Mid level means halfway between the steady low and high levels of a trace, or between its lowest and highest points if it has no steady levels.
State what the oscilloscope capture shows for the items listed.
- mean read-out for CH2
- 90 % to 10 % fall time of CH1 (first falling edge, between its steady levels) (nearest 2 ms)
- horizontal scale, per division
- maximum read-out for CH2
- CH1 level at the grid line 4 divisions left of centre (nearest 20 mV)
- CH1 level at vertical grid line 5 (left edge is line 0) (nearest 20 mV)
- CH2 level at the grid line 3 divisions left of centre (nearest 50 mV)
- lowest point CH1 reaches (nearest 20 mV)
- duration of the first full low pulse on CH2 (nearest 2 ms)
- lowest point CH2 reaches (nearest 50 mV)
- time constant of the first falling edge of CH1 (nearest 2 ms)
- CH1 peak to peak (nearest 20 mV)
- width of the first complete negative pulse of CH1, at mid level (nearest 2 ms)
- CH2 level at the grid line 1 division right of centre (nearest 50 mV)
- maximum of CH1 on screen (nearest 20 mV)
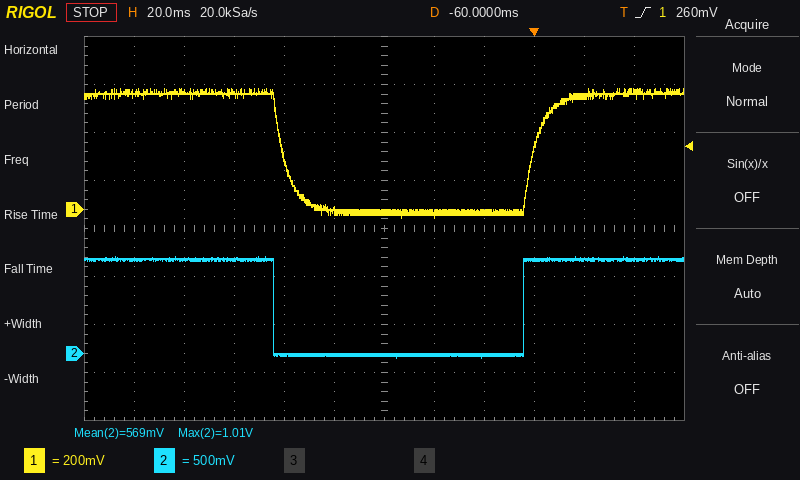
569 mV
12 ms
20 ms
1.01 V
500 mV
0 mV
1.00 V
-40 mV
100 ms
-50 mV
6 ms
540 mV
100 ms
0 mV
500 mV
